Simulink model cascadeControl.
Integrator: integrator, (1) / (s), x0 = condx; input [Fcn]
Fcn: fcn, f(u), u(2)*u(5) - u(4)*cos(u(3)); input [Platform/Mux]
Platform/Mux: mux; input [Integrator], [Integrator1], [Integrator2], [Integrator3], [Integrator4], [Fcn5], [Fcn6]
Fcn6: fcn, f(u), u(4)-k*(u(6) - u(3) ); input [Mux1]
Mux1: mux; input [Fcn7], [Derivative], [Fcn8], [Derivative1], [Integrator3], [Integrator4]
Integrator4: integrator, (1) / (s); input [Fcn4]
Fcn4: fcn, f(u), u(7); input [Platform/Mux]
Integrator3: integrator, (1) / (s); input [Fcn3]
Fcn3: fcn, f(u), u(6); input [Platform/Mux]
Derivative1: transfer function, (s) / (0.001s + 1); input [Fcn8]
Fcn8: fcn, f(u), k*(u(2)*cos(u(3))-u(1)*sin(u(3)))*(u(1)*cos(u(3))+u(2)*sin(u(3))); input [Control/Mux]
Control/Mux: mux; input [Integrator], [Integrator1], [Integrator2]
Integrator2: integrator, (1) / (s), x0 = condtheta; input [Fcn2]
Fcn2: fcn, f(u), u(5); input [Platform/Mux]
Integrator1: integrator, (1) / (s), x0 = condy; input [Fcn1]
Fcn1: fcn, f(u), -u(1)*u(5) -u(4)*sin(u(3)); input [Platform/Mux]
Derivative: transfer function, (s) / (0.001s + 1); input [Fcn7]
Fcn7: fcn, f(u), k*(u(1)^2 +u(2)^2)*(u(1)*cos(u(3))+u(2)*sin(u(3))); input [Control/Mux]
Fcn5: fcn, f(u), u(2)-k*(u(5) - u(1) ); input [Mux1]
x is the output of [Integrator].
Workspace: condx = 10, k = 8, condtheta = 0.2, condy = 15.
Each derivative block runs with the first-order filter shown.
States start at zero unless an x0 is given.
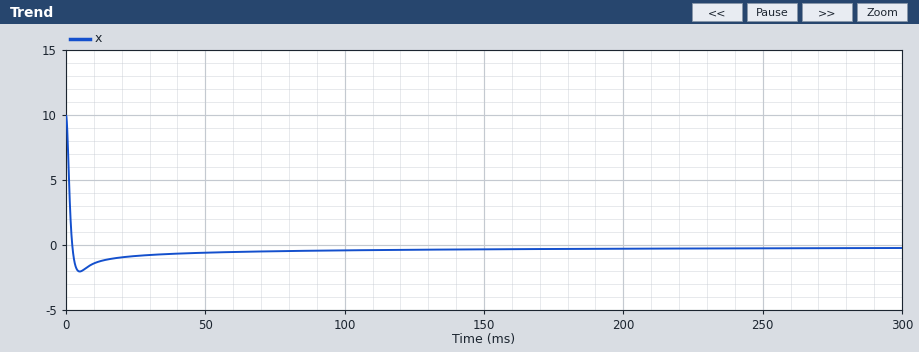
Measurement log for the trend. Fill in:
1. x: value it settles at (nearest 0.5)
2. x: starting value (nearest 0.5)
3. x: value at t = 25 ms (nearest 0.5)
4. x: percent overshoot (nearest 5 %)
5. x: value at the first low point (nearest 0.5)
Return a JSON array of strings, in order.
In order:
["0.0", "10.0", "-1.0", "20 %", "-2.0"]
